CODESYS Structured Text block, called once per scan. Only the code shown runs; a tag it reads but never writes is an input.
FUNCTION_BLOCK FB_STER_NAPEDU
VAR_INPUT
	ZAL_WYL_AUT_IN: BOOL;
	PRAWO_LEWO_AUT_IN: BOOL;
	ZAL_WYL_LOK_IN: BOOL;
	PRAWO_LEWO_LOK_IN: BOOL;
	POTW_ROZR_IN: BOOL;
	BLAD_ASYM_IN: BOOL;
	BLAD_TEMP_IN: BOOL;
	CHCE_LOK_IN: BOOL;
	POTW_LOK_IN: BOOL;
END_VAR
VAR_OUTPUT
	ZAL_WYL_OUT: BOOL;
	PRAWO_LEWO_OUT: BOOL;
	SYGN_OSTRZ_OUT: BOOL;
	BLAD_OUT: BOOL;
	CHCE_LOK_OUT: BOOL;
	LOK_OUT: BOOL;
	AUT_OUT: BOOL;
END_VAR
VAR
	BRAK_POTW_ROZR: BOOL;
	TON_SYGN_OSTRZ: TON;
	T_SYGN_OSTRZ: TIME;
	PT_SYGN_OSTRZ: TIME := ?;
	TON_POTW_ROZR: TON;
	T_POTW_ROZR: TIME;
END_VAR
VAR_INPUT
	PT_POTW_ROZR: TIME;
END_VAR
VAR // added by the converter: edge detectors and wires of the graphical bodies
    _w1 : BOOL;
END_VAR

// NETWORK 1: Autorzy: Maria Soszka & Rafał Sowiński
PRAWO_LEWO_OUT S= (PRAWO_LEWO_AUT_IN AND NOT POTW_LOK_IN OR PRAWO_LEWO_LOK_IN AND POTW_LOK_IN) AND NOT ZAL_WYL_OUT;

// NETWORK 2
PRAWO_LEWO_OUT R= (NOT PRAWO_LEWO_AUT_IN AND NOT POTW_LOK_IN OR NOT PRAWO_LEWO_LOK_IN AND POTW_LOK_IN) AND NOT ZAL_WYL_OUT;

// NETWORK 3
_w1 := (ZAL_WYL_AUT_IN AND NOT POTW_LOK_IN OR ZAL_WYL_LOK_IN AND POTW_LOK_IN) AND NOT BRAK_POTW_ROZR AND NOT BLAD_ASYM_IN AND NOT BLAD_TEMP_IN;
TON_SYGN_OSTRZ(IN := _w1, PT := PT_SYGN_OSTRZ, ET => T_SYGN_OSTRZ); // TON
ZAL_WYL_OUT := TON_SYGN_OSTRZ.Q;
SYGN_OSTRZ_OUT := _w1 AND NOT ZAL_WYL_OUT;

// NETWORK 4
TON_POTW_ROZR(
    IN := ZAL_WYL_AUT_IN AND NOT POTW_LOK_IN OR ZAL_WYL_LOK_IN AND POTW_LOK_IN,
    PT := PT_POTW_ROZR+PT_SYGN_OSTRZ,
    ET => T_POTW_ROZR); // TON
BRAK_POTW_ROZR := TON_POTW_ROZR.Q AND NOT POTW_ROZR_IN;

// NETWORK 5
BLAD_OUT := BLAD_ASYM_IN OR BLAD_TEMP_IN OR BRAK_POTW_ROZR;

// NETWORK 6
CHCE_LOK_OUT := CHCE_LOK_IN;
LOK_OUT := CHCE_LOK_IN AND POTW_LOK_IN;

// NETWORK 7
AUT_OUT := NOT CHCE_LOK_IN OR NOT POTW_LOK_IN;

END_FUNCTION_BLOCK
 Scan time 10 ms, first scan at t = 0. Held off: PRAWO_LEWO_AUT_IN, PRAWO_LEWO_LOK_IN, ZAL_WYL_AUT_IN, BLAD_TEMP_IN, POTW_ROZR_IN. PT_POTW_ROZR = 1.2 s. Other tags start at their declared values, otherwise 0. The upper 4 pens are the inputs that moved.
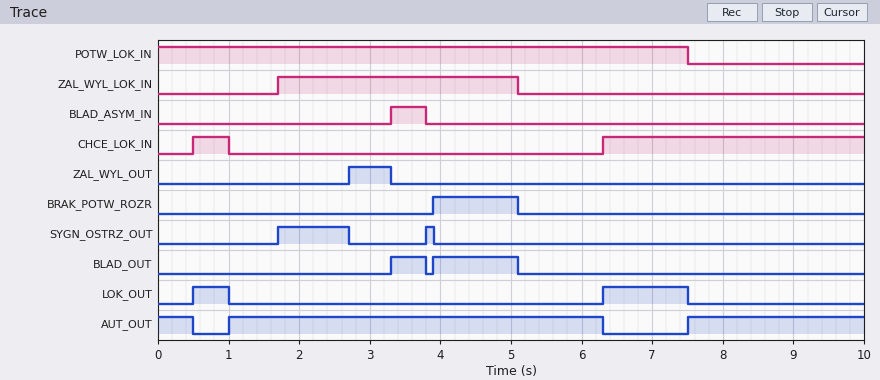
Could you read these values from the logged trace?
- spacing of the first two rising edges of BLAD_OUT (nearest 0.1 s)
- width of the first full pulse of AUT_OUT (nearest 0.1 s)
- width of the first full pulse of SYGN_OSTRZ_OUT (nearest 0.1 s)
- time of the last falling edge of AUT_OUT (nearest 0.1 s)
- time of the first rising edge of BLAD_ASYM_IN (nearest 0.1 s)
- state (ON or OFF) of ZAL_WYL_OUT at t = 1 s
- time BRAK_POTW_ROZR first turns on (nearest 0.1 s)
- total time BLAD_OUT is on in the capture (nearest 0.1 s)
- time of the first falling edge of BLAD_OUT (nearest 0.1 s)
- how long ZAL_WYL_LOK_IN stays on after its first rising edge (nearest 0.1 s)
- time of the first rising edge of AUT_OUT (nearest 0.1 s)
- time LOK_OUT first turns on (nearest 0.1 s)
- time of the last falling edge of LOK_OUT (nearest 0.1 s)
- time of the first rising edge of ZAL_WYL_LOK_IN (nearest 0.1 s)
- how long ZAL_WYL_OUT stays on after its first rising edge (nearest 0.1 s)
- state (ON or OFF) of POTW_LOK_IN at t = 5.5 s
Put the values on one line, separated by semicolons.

0.6 s; 5.3 s; 1.0 s; 6.3 s; 3.3 s; OFF; 3.9 s; 1.7 s; 3.8 s; 3.4 s; 1.0 s; 0.5 s; 7.5 s; 1.7 s; 0.6 s; ON
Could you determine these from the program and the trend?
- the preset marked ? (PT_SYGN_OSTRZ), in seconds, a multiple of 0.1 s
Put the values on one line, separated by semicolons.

1.0 s
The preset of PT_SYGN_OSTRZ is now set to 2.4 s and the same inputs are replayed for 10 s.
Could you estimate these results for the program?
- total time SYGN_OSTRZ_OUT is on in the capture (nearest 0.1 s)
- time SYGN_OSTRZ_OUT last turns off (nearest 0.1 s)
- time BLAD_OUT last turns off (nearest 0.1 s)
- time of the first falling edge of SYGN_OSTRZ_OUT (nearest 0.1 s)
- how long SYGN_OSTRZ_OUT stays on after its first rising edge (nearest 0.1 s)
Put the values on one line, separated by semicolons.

2.9 s; 5.1 s; 3.8 s; 3.3 s; 1.6 s
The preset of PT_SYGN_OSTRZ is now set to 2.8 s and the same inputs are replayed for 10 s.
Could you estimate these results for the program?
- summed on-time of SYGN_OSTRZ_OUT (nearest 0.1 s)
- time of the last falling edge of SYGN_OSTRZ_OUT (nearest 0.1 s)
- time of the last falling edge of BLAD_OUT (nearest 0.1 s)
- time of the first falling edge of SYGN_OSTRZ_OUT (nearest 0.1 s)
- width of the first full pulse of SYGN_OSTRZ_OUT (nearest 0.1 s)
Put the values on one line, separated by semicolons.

2.9 s; 5.1 s; 3.8 s; 3.3 s; 1.6 s
